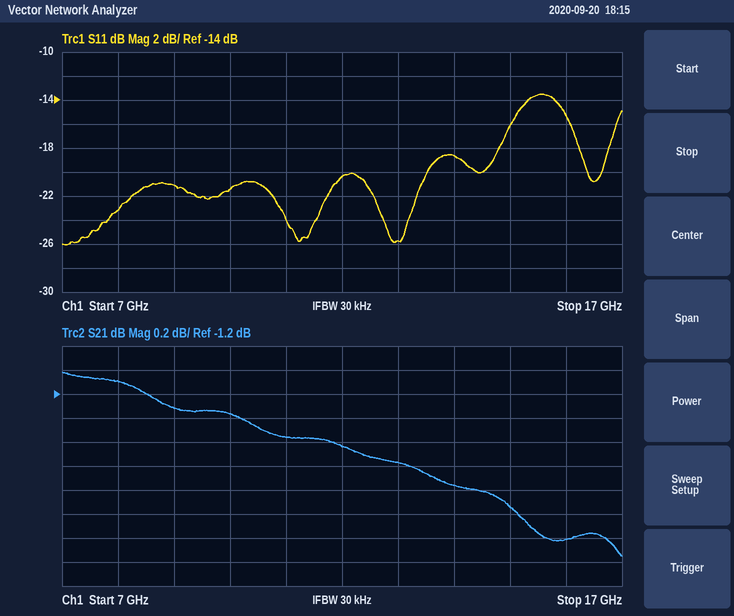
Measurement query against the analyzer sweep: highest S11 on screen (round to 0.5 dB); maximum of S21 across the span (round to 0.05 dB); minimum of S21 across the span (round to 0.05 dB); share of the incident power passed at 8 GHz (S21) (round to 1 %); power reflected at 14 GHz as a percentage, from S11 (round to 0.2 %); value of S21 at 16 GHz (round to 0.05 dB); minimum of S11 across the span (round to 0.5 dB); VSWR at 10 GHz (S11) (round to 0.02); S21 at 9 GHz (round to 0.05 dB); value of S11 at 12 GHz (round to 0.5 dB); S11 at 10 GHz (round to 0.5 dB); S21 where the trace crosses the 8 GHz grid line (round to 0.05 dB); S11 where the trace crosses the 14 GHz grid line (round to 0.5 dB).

-13.5 dB
-1.00 dB
-2.55 dB
78 %
1.4 %
-2.40 dB
-26.0 dB
1.18
-1.30 dB
-20.5 dB
-21.5 dB
-1.10 dB
-18.5 dB
